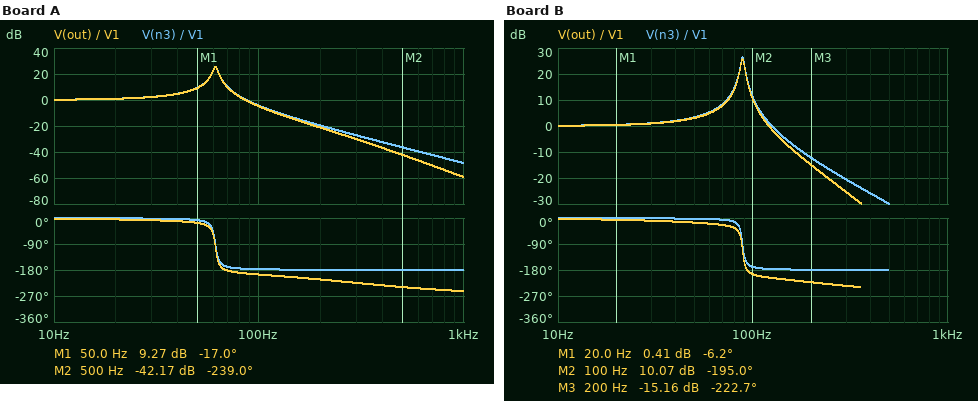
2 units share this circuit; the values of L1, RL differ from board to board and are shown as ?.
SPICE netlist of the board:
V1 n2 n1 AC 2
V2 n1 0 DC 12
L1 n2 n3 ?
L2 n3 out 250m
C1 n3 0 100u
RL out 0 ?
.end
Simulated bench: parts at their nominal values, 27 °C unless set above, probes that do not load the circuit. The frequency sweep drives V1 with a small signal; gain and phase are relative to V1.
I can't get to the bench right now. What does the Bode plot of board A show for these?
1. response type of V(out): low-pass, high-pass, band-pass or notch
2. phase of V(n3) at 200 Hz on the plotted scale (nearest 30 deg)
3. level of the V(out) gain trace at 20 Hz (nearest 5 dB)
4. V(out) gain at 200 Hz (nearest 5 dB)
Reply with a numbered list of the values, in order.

1. low-pass
2. -180 deg
3. 0 dB
4. -20 dB
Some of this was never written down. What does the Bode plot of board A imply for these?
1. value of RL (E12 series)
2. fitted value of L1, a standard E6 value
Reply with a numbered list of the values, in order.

1. 470 Ω
2. 68 mH
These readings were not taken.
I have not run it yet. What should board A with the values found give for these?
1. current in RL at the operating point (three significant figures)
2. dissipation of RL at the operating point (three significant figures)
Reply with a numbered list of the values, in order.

1. 25.5 mA
2. 306 mW
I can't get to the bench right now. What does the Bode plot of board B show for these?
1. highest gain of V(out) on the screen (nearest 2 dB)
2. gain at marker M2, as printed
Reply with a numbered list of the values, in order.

1. 26 dB
2. 10.07 dB
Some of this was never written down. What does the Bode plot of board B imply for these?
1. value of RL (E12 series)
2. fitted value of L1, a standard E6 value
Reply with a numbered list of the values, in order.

1. 330 Ω
2. 33 mH
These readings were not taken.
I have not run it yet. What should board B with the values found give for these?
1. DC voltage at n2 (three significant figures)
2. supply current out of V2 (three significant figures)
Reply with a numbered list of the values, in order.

1. 12.0 V
2. 36.4 mA
